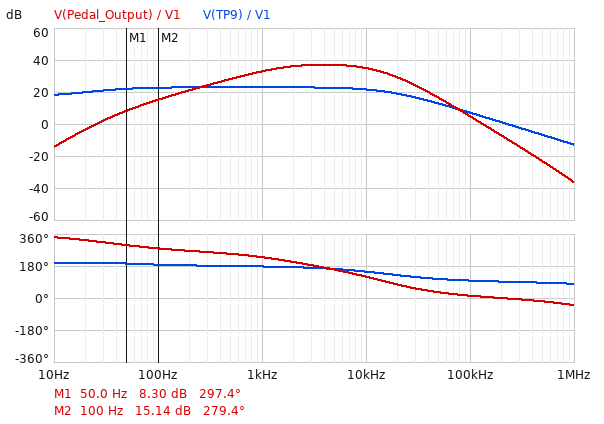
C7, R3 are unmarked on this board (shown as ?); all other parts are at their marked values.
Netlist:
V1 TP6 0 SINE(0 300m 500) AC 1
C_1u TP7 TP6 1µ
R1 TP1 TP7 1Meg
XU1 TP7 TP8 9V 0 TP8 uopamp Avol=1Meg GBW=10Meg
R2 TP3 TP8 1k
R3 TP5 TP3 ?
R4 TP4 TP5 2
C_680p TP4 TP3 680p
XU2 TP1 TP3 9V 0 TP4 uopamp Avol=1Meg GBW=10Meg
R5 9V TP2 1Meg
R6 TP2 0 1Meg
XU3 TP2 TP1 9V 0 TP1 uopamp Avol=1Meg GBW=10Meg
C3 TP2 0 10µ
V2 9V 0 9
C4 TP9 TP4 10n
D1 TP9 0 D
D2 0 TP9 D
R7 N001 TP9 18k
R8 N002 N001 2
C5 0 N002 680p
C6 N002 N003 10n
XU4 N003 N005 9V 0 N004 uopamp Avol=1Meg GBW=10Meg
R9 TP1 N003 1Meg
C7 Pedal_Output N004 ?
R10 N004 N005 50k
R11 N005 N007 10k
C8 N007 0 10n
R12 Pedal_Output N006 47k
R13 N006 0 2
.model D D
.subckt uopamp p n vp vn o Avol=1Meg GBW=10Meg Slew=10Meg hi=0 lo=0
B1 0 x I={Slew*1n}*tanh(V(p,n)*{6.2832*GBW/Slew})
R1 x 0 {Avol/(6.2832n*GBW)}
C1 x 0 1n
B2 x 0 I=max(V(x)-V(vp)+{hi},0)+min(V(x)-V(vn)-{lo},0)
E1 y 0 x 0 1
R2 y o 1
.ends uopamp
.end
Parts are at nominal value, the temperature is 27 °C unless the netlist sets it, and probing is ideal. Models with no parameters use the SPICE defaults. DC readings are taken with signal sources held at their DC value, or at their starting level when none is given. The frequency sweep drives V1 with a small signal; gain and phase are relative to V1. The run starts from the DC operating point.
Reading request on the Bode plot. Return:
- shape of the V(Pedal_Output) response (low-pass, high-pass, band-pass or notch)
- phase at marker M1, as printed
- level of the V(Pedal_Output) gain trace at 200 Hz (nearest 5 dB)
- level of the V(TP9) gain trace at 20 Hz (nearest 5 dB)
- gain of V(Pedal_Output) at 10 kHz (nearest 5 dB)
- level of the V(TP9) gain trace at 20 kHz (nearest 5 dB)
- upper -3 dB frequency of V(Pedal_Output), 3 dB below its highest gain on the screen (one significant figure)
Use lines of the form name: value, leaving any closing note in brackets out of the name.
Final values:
shape of the V(Pedal_Output) response: band-pass
phase at marker M1, as printed: 297.4 deg
level of the V(Pedal_Output) gain trace at 200 Hz: 20 dB
level of the V(TP9) gain trace at 20 Hz: 20 dB
gain of V(Pedal_Output) at 10 kHz: 35 dB
level of the V(TP9) gain trace at 20 kHz: 20 dB
upper -3 dB frequency of V(Pedal_Output), 3 dB below its highest gain on the screen: 10 kHz
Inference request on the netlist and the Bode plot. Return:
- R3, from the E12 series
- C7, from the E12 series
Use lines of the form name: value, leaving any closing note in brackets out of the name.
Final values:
R3, from the E12 series: 15 kΩ
C7, from the E12 series: 15 nF
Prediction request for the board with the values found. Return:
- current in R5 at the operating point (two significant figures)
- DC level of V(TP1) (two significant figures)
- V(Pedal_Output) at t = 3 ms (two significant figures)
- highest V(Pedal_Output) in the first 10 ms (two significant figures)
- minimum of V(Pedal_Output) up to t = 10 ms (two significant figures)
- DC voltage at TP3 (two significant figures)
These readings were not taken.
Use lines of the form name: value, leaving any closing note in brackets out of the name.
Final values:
current in R5 at the operating point: 4.5 µA
DC level of V(TP1): 4.5 V
V(Pedal_Output) at t = 3 ms: 380 mV
highest V(Pedal_Output) in the first 10 ms: 3.2 V
minimum of V(Pedal_Output) up to t = 10 ms: -3.2 V
DC voltage at TP3: 4.5 V
